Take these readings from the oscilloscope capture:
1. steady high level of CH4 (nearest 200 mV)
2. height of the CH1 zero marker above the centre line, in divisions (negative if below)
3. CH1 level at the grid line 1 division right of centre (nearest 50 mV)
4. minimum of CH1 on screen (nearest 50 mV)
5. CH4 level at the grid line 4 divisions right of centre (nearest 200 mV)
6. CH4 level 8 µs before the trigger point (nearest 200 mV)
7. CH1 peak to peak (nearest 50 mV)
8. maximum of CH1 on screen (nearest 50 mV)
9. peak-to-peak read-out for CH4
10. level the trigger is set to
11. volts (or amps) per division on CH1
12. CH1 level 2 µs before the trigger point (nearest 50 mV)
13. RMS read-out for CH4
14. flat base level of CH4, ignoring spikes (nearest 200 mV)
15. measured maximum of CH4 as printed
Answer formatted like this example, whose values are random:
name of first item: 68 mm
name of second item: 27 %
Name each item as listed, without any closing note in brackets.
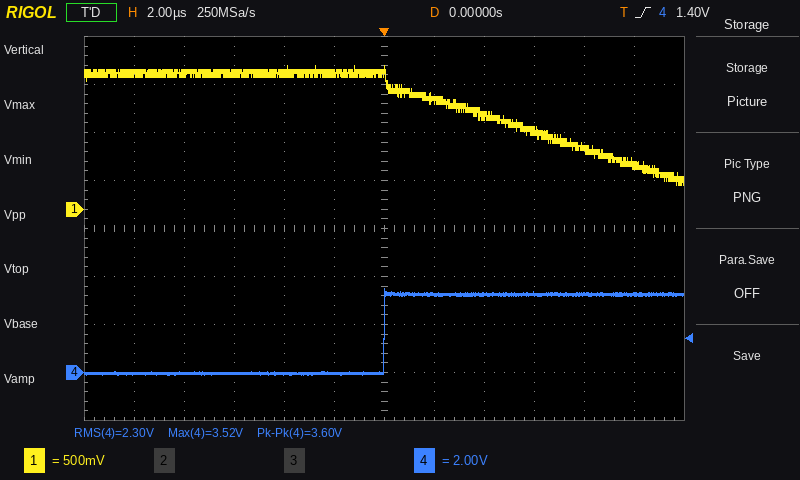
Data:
steady high level of CH4: 3.2 V
height of the CH1 zero marker above the centre line, in divisions: +0.4 div
CH1 level at the grid line 1 division right of centre: 1.15 V
minimum of CH1 on screen: 250 mV
CH4 level at the grid line 4 divisions right of centre: 3.2 V
CH4 level 8 µs before the trigger point: 0.0 V
CH1 peak to peak: 1.25 V
maximum of CH1 on screen: 1.50 V
peak-to-peak read-out for CH4: 3.60 V
level the trigger is set to: 1.40 V
volts (or amps) per division on CH1: 500 mV
CH1 level 2 µs before the trigger point: 1.40 V
RMS read-out for CH4: 2.30 V
flat base level of CH4, ignoring spikes: 0.0 V
measured maximum of CH4 as printed: 3.52 V
